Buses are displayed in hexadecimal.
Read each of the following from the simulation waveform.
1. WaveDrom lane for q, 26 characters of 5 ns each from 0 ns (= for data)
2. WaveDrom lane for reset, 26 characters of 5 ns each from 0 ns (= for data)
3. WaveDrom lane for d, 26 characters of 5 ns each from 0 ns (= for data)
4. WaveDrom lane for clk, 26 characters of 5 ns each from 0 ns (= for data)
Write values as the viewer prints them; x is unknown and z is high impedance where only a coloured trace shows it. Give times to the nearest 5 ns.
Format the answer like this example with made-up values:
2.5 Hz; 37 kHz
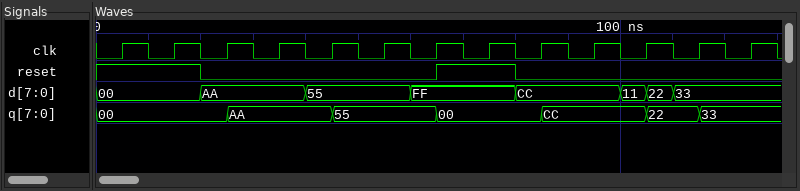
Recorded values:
{name: 'q', wave: '=....=...=...=...=...=.=..', data: '00 AA 55 00 CC 22 33'}; {name: 'reset', wave: '1...0........1..0.........'}; {name: 'd', wave: '=...=...=...=...=...===...', data: '00 AA 55 FF CC 11 22 33'}; {name: 'clk', wave: '01010101010101010101010101'}
